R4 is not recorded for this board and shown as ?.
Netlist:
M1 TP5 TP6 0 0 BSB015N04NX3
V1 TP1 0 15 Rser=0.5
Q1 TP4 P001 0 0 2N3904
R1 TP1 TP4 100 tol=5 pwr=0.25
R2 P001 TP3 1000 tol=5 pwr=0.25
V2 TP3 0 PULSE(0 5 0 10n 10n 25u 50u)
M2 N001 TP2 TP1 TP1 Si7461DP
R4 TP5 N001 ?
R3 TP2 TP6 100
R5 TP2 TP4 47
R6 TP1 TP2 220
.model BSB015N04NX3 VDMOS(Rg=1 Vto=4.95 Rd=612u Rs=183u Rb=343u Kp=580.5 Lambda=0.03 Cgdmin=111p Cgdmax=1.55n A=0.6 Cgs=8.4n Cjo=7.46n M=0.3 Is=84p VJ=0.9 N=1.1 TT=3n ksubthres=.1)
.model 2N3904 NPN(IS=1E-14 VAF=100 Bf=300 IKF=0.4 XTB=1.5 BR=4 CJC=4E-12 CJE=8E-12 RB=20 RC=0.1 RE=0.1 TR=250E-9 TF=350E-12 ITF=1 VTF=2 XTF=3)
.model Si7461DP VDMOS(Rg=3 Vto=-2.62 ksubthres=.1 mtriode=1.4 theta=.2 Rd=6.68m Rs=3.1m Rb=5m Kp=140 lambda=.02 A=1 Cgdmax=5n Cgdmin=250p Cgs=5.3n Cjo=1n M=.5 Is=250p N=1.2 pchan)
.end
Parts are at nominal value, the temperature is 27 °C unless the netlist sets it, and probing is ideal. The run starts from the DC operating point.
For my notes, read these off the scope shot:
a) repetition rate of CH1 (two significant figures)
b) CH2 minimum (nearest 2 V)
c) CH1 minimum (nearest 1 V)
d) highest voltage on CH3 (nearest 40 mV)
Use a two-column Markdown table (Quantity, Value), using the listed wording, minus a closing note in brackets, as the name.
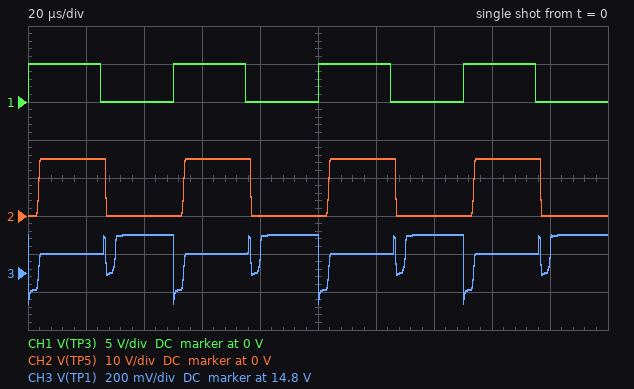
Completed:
| Quantity | Value |
|---|---|
| repetition rate of CH1 | 20 kHz |
| CH2 minimum | 0 V |
| CH1 minimum | 0 V |
| highest voltage on CH3 | 15.00 V |
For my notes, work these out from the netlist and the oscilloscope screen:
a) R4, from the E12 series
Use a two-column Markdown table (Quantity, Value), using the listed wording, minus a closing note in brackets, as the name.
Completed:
| Quantity | Value |
|---|---|
| R4, from the E12 series | 39 Ω |
